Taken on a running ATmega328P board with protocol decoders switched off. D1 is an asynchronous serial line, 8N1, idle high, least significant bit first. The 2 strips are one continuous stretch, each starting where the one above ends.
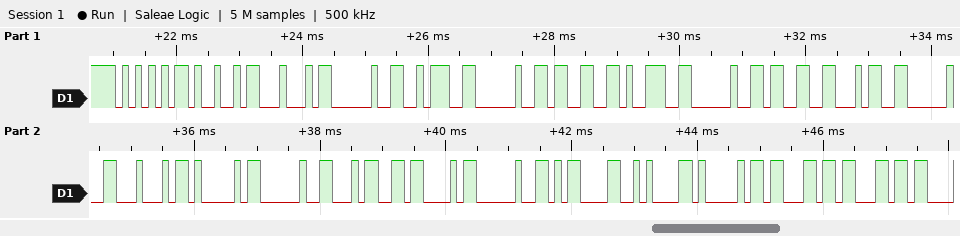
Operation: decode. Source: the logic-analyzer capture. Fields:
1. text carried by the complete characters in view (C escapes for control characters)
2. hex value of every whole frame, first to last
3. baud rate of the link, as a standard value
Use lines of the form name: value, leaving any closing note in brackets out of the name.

text carried by the complete characters in view: "UID : 39 34 DA 4C \r\nAcc"
hex value of every whole frame, first to last: 55 49 44 20 3A 20 33 39 20 33 34 20 44 41 20 34 43 20 0D 0A 41 63 63
baud rate of the link, as a standard value: 9600 baud
